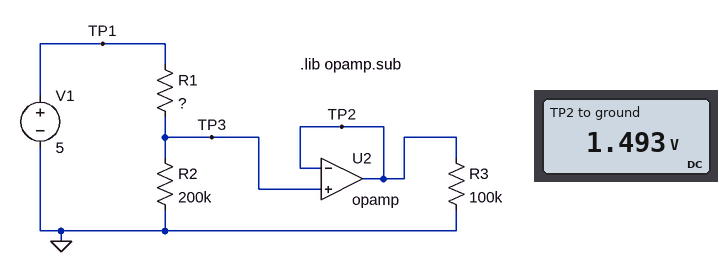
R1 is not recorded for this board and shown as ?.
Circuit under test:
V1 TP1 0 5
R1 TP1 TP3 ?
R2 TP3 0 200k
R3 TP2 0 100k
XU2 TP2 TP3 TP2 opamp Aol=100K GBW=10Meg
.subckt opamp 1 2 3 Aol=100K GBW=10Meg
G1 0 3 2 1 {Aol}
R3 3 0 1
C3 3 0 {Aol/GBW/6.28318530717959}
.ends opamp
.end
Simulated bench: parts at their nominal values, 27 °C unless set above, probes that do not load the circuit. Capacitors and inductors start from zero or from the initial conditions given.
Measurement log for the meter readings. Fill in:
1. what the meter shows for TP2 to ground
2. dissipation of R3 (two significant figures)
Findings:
1.493 V
22 µW
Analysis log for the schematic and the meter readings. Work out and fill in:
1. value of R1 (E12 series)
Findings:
470 kΩ
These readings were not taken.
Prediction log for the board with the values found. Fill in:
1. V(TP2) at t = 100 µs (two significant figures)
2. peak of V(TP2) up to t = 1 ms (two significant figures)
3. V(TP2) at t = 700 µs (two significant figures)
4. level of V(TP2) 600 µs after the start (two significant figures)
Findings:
1.5 V
1.5 V
1.5 V
1.5 V
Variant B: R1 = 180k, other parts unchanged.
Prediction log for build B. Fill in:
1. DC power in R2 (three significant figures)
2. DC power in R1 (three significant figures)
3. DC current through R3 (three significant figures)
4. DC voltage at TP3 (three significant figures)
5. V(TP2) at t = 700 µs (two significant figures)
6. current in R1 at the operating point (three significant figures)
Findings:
34.6 µW
31.2 µW
26.3 µA
2.63 V
2.6 V
13.2 µA
